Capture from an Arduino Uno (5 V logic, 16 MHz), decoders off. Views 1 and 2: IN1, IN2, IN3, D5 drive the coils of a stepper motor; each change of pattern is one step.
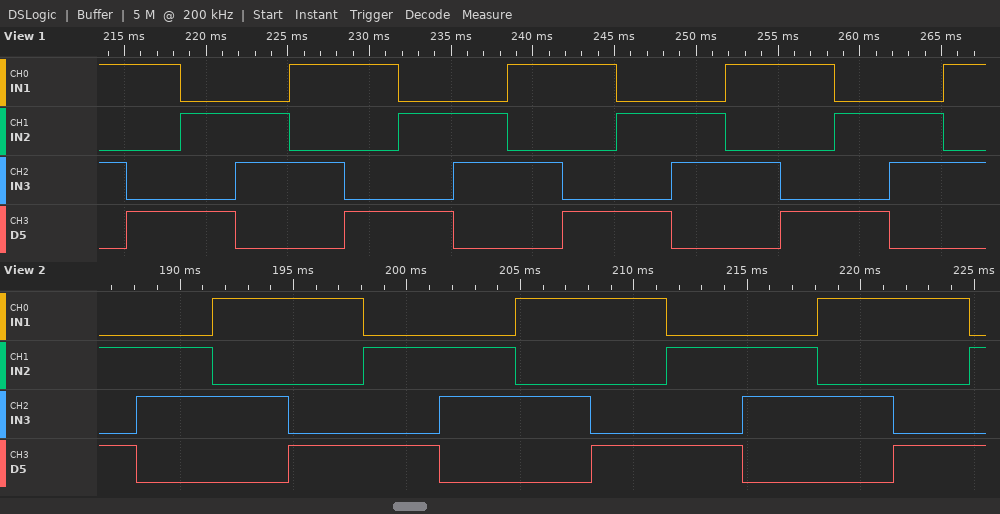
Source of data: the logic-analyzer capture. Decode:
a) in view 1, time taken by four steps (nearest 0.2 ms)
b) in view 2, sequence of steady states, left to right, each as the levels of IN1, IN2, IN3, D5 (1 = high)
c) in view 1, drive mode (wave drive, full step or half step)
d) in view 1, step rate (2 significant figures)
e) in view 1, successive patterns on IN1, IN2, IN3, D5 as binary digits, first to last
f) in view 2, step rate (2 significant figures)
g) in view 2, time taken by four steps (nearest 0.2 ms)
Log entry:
13.4 ms
0101 0110 1010 1001 0101 0110 1010 1001 0101 0110 1010 1001 0101
full step
300 steps/s
1010 1001 0101 0110 1010 1001 0101 0110 1010 1001 0101 0110 1010 1001 0101 0110 1010
300 steps/s
13.4 ms
